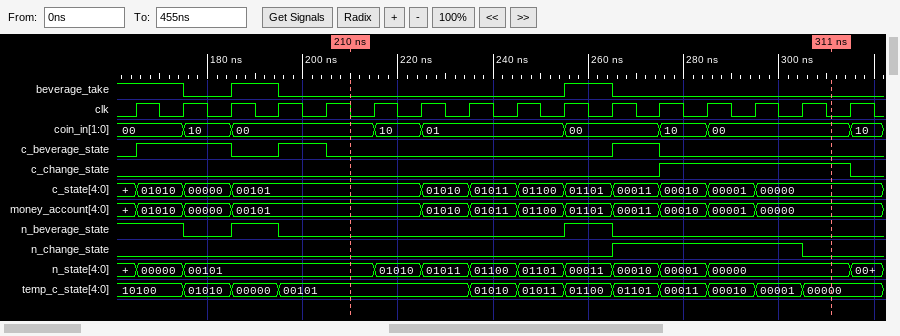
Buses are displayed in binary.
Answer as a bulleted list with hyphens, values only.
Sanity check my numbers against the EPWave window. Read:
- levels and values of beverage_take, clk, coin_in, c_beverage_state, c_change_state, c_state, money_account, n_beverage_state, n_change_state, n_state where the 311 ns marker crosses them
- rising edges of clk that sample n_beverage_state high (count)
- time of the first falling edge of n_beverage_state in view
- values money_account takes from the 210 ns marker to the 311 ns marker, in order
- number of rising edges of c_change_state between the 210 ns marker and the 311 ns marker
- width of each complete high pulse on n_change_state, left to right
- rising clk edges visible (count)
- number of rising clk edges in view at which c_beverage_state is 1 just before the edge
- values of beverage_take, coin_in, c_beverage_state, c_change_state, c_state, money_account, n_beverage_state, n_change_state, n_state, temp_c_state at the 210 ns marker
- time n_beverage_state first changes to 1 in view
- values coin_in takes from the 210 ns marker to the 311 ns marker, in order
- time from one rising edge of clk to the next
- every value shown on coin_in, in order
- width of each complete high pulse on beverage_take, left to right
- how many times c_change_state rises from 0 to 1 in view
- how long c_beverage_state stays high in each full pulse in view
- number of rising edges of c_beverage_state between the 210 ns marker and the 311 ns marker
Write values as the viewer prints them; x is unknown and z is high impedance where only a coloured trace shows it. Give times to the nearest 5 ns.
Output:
- beverage_take=0, clk=0, coin_in=00, c_beverage_state=0, c_change_state=1, c_state=00000, money_account=00000, n_beverage_state=0, n_change_state=0, n_state=00000
- 4
- 175 ns
- 00101, 01010, 01011, 01100, 01101, 00011, 00010, 00001, 00000
- 1
- 40 ns
- 16
- 4
- beverage_take=0, coin_in=00, c_beverage_state=0, c_change_state=0, c_state=00101, money_account=00101, n_beverage_state=0, n_change_state=0, n_state=00101, temp_c_state=00101
- 185 ns
- 00, 10, 01, 00, 10, 00
- 10 ns
- 00, 10, 00, 10, 01, 00, 10, 00, 10
- 10 ns, 10 ns
- 1
- 20 ns, 10 ns, 10 ns
- 1
